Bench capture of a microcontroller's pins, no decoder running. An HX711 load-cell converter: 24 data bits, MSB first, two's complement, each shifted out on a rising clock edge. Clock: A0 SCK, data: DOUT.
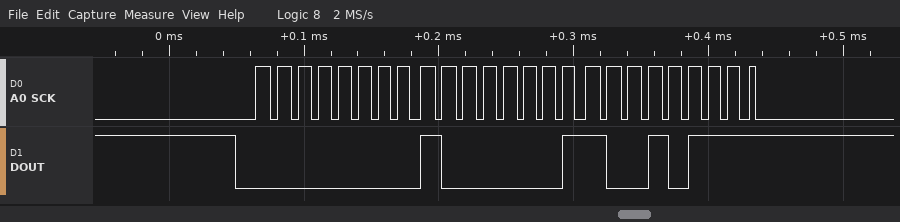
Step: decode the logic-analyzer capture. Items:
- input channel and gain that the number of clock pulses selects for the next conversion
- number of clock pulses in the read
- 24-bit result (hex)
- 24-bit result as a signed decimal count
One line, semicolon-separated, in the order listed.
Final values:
channel A, gain 128; 25; 0x008197; 33175
